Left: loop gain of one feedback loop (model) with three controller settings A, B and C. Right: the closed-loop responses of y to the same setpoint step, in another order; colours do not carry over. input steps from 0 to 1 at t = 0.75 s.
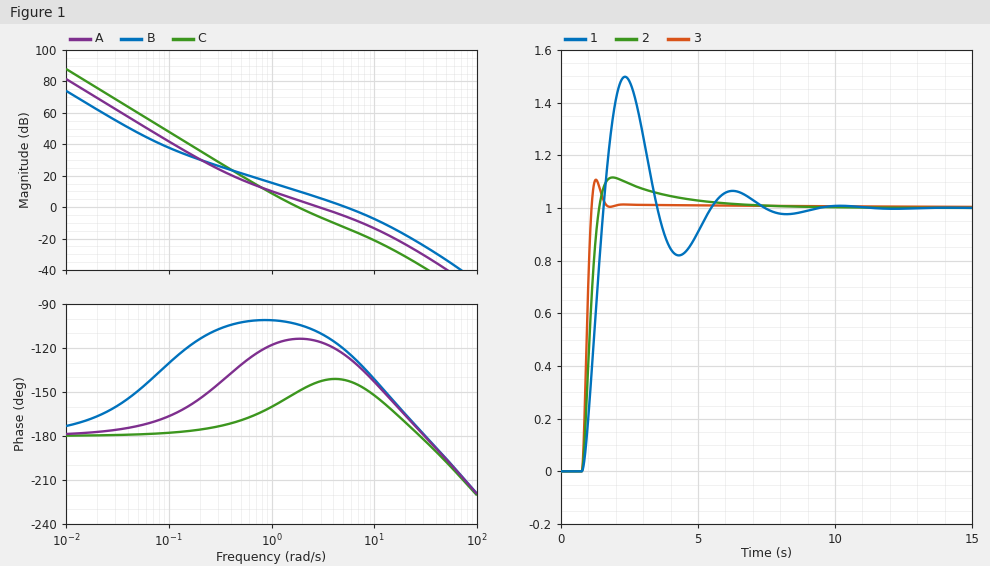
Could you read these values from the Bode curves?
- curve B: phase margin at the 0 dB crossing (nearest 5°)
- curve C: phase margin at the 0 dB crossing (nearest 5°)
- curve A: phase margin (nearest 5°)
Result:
60°
30°
65°
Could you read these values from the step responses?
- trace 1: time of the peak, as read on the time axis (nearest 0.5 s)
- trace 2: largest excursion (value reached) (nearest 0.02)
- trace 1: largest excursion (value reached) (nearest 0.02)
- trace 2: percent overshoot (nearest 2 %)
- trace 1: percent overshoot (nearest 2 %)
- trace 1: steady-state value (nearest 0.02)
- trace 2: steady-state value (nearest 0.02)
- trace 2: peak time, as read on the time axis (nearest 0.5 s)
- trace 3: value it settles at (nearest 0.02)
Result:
2.5 s
1.12
1.50
12 %
50 %
1.00
1.00
2.0 s
1.00
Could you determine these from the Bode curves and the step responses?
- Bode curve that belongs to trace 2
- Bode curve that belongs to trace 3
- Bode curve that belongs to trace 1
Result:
A
B
C
